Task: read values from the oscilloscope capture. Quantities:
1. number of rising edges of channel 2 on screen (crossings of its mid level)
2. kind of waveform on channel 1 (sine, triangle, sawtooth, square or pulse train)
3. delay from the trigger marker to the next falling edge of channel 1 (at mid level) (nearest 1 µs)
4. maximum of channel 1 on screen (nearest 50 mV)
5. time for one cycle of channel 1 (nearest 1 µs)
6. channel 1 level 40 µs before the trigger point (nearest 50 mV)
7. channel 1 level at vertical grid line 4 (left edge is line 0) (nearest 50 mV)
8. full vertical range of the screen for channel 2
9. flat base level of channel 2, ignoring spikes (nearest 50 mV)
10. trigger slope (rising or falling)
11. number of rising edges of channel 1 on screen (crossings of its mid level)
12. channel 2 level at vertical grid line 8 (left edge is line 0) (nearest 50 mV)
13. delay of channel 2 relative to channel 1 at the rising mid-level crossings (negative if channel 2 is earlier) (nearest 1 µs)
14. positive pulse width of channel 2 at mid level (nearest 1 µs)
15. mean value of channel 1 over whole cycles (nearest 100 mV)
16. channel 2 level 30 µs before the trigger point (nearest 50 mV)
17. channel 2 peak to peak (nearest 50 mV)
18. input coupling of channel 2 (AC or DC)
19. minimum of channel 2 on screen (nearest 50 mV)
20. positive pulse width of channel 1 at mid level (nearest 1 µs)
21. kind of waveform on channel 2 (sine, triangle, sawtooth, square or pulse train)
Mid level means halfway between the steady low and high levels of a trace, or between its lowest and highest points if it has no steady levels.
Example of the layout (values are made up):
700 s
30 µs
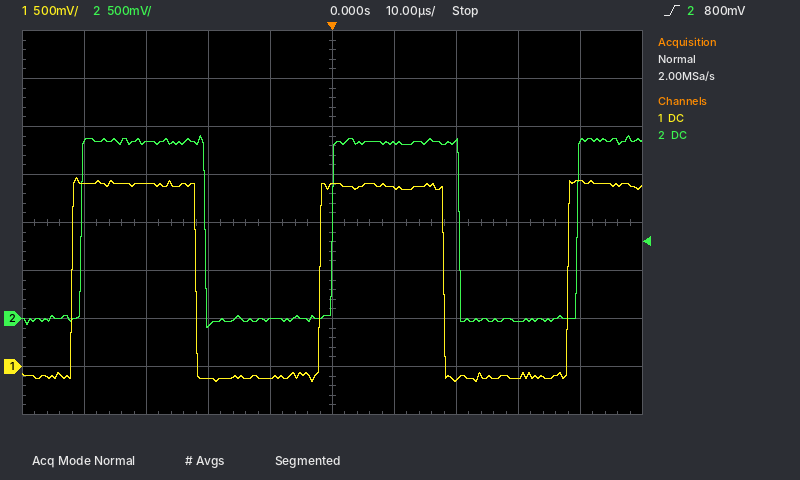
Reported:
3
square
18 µs
1.95 V
40 µs
1.90 V
-100 mV
4 V
0 mV
rising
3
-50 mV
+2 µs
20 µs
900 mV
1.85 V
2.00 V
DC
-100 mV
20 µs
square
